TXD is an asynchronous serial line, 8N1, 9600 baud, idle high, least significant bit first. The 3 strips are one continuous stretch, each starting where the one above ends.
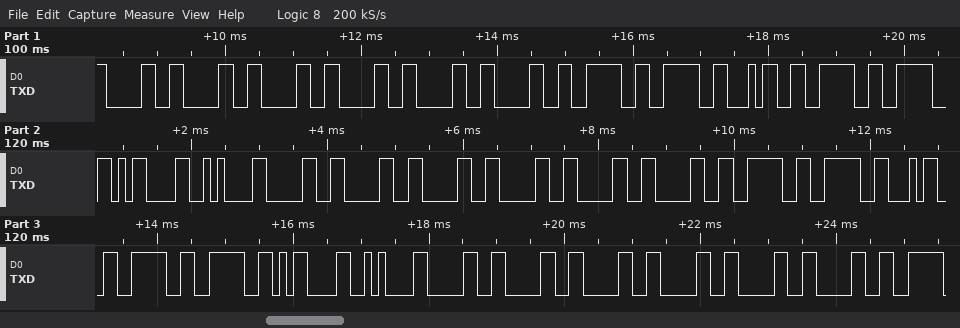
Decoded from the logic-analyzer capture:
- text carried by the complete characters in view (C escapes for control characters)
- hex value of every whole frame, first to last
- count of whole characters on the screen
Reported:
"000000>>4>>\r\n000000>>4>>\r\n000000"
30 30 30 30 30 30 3E 3E 34 3E 3E 0D 0A 30 30 30 30 30 30 3E 3E 34 3E 3E 0D 0A 30 30 30 30 30 30
32
